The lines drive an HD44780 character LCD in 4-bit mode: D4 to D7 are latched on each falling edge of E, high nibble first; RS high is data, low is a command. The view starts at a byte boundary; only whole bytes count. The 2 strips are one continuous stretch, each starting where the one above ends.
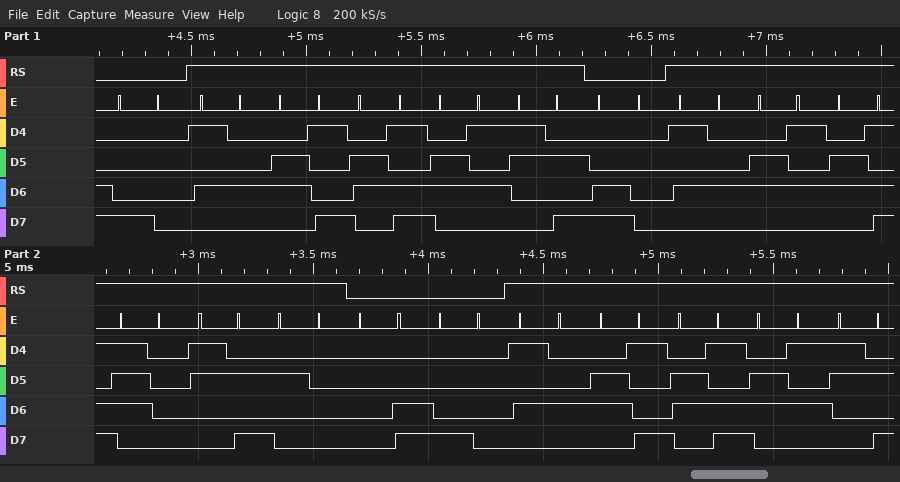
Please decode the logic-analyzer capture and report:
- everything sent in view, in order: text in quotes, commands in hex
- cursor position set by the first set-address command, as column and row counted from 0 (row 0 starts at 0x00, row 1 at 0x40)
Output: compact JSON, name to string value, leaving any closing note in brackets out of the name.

{"everything sent in view, in order: text in quotes, commands in hex": "0x80 \"Time:\" 0xC0 \"Temp: \" 0x0C 0x80 \"Time:\"", "cursor position set by the first set-address command, as column and row counted from 0": "column 0, row 0"}
